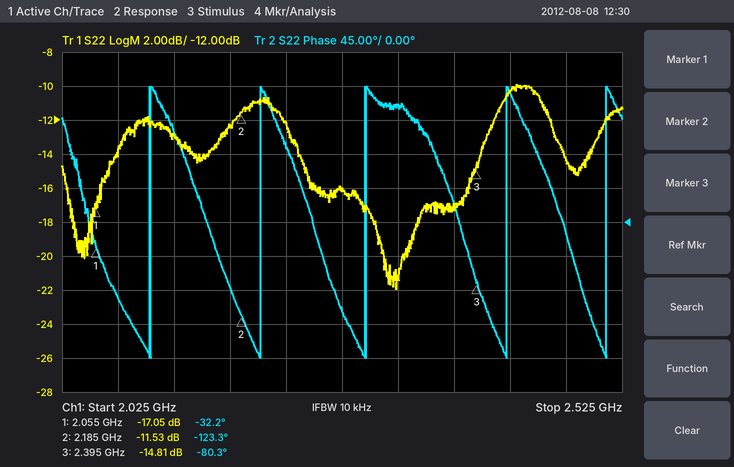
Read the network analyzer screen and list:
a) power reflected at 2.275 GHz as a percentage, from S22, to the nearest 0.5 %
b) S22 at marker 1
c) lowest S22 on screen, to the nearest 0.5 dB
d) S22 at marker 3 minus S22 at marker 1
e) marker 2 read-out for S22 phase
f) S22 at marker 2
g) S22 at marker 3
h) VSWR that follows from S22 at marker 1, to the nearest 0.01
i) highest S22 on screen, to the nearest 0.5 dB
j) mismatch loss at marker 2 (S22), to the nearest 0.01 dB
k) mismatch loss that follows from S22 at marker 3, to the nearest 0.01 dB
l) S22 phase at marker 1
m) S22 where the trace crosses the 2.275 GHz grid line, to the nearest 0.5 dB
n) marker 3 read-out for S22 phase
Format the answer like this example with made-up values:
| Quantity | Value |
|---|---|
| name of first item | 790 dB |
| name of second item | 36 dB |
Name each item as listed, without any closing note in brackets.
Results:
| Quantity | Value |
|---|---|
| power reflected at 2.275 GHz as a percentage, from S22, to the nearest 0.5 % | 2.5 % |
| S22 at marker 1 | -17.05 dB |
| lowest S22 on screen, to the nearest 0.5 dB | -22.0 dB |
| S22 at marker 3 minus S22 at marker 1 | 2.24 dB |
| marker 2 read-out for S22 phase | -123.3° |
| S22 at marker 2 | -11.53 dB |
| S22 at marker 3 | -14.81 dB |
| VSWR that follows from S22 at marker 1, to the nearest 0.01 | 1.33 |
| highest S22 on screen, to the nearest 0.5 dB | -10.0 dB |
| mismatch loss at marker 2 (S22), to the nearest 0.01 dB | 0.32 dB |
| mismatch loss that follows from S22 at marker 3, to the nearest 0.01 dB | 0.15 dB |
| S22 phase at marker 1 | -32.2° |
| S22 where the trace crosses the 2.275 GHz grid line, to the nearest 0.5 dB | -16.0 dB |
| marker 3 read-out for S22 phase | -80.3° |
